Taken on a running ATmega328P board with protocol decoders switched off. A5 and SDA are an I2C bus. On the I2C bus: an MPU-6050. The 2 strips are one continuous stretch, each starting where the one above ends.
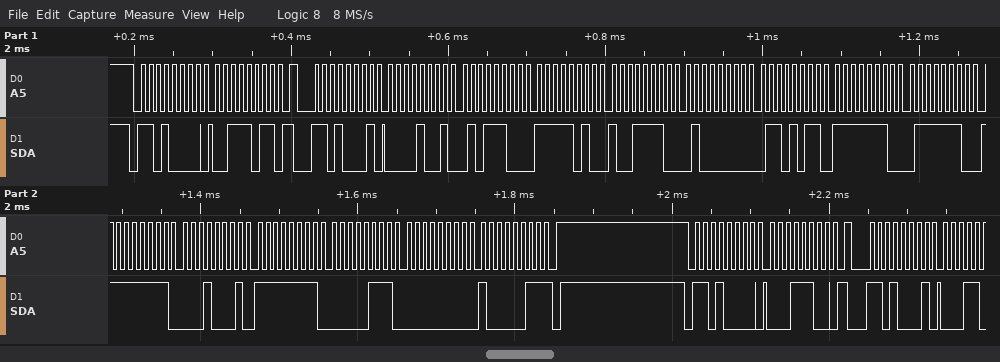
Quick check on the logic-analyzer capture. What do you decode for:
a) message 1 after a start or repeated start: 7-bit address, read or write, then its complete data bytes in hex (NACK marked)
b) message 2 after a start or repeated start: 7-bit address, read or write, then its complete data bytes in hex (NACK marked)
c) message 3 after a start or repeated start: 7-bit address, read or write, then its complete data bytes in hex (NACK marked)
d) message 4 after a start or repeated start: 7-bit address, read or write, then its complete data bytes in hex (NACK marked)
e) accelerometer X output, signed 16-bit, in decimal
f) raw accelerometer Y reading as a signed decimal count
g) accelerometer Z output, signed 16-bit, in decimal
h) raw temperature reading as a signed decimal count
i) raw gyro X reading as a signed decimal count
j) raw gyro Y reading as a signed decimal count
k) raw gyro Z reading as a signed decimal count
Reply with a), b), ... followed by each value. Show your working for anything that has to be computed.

a) 0x68 write: 3B
b) 0x68 read: 09 5C FA 9E 40 6B FE 7E FF 11 FF 07 00 83 NACK
c) 0x68 write: 1C
d) 0x68 read
e) 0x095C = 2396
f) 0xFA9E = -1378
g) 0x406B = 16491
h) 0xFE7E = -386
i) 0xFF11 = -239
j) 0xFF07 = -249
k) 0x0083 = 131
